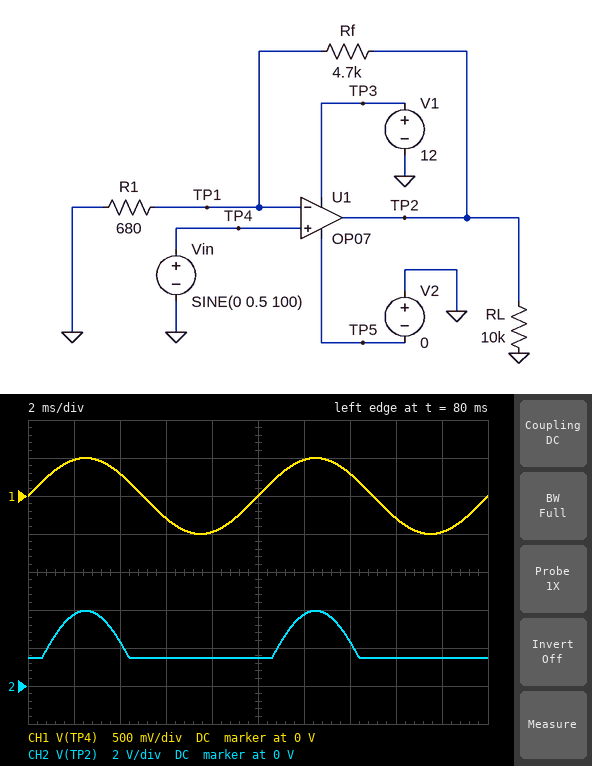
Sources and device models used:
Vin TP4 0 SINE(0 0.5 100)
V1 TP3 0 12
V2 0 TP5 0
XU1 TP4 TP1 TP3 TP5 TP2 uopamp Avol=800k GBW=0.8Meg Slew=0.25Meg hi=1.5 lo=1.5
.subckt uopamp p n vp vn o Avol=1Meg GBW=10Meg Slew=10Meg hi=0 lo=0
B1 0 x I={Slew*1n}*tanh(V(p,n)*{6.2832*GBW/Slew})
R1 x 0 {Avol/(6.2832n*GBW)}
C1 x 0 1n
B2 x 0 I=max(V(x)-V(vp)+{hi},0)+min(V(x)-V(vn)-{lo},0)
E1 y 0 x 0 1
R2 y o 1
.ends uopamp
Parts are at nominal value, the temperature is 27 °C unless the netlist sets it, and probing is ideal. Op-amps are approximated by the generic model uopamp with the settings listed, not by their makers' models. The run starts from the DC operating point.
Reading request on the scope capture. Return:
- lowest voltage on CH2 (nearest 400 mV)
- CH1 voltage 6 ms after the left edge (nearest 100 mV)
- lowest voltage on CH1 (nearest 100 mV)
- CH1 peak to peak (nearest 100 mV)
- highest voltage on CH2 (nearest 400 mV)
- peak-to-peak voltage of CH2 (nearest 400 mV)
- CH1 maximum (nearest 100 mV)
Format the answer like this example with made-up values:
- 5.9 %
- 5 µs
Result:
- 1.6 V
- -300 mV
- -500 mV
- 1.0 V
- 4.0 V
- 2.4 V
- 500 mV
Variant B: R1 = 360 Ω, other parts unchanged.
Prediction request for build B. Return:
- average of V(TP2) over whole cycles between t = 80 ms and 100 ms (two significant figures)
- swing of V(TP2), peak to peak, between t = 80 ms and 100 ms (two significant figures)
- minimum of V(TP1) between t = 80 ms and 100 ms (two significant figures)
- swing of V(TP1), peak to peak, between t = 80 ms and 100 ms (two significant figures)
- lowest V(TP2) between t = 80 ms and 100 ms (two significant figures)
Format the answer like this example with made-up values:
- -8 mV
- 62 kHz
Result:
- 3.0 V
- 5.5 V
- 110 mV
- 390 mV
- 1.5 V
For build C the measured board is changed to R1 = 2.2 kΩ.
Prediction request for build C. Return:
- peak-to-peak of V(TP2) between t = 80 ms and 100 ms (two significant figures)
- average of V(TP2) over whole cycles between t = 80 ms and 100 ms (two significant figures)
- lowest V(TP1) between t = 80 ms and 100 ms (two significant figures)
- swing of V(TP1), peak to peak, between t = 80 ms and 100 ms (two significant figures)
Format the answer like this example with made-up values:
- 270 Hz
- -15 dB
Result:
- 69 mV
- 1.5 V
- 480 mV
- 22 mV
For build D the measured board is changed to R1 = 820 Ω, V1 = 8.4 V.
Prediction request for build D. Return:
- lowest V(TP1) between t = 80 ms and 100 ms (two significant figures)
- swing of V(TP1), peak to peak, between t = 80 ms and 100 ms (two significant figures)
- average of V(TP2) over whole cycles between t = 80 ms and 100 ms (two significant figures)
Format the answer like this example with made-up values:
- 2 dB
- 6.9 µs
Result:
- 220 mV
- 280 mV
- 1.9 V
